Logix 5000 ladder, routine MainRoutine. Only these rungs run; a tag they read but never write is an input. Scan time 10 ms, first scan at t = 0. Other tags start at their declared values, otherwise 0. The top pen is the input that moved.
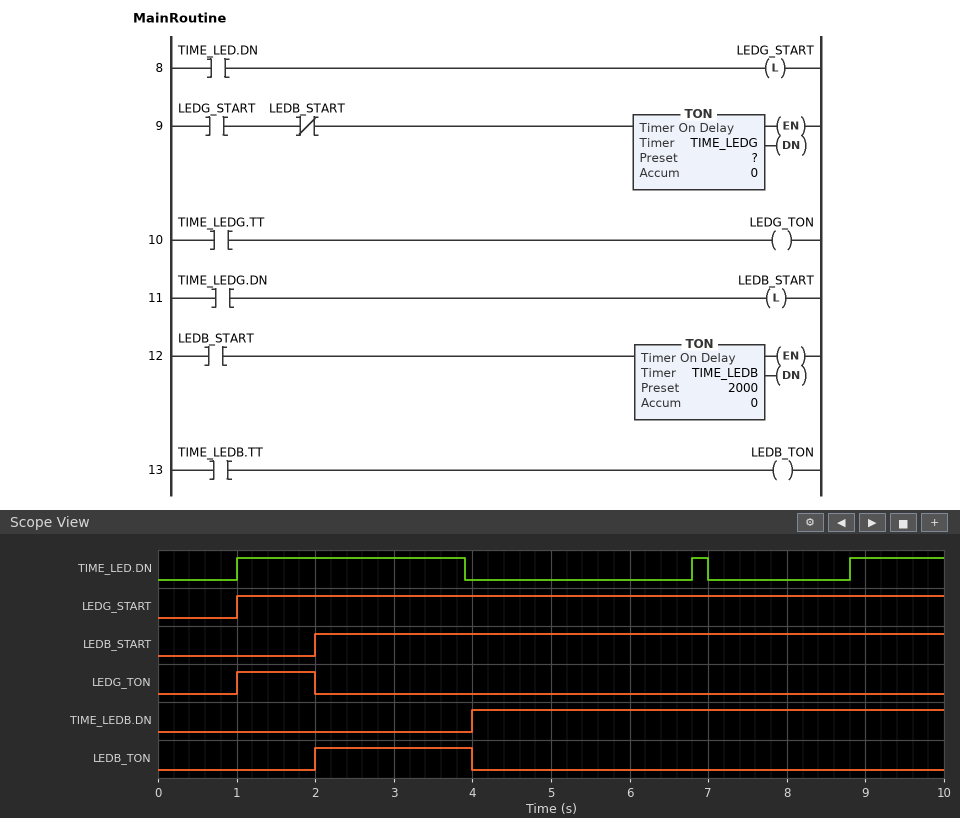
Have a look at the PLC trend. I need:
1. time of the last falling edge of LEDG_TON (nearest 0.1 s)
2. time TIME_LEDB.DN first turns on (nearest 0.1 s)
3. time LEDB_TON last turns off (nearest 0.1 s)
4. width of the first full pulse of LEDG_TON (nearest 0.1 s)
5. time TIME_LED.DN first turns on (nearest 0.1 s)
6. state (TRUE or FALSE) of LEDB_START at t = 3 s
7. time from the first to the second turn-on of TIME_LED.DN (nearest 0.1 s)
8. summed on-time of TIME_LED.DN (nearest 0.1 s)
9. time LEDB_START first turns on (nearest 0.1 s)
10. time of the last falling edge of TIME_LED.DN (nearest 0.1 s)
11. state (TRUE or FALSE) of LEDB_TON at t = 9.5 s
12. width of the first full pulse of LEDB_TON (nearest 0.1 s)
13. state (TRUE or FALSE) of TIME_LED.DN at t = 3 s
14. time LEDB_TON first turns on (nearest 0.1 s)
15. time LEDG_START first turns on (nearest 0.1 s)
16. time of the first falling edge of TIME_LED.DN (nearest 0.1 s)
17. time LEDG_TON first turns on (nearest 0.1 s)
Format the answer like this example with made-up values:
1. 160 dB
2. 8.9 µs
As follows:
1. 2.0 s
2. 4.0 s
3. 4.0 s
4. 1.0 s
5. 1.0 s
6. TRUE
7. 5.8 s
8. 4.3 s
9. 2.0 s
10. 7.0 s
11. FALSE
12. 2.0 s
13. TRUE
14. 2.0 s
15. 1.0 s
16. 3.9 s
17. 1.0 s
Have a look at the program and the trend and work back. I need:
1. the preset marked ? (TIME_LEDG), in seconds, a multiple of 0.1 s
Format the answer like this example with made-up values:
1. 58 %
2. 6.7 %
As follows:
1. 1.0 s
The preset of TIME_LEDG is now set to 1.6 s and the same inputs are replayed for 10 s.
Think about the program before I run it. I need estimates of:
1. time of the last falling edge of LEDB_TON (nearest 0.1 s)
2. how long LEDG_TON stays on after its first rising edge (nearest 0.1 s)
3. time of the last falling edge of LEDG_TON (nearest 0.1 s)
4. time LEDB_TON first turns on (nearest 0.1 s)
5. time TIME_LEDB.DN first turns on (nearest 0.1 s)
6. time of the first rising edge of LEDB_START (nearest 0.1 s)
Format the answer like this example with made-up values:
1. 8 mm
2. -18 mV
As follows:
1. 4.6 s
2. 1.6 s
3. 2.6 s
4. 2.6 s
5. 4.6 s
6. 2.6 s
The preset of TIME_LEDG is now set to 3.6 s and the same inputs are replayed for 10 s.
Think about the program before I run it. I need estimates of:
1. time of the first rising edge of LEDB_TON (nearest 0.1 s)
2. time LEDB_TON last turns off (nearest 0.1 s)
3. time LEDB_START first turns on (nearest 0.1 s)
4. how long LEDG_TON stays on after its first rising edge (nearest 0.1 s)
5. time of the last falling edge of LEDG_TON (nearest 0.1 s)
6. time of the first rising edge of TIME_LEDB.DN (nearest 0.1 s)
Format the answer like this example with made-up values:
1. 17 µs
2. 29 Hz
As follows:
1. 4.6 s
2. 6.6 s
3. 4.6 s
4. 3.6 s
5. 4.6 s
6. 6.6 s
